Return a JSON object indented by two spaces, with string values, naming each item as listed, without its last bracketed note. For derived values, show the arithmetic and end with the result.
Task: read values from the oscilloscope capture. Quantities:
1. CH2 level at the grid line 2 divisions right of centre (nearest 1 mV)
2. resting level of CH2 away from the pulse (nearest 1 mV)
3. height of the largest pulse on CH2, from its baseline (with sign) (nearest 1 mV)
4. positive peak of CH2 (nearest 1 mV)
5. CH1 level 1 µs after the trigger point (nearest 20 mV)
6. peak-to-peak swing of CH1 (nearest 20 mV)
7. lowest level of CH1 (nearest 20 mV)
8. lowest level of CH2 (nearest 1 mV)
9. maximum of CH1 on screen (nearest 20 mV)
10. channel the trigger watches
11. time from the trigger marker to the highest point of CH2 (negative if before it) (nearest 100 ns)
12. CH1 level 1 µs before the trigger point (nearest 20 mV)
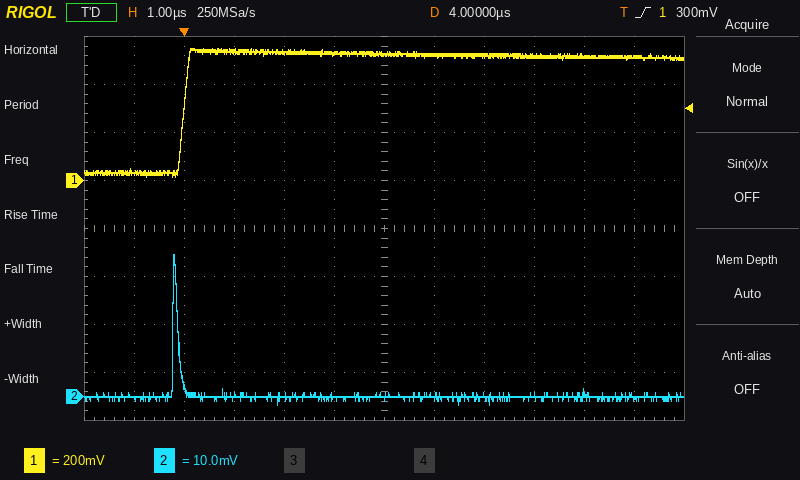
{
  "CH2 level at the grid line 2 divisions right of centre": "0 mV",
  "resting level of CH2 away from the pulse": "0 mV",
  "height of the largest pulse on CH2, from its baseline (with sign)": "30 mV − (0 mV) = +30 mV",
  "positive peak of CH2": "30 mV",
  "CH1 level 1 µs after the trigger point": "540 mV",
  "peak-to-peak swing of CH1": "560 mV − (20 mV) = 540 mV",
  "lowest level of CH1": "20 mV",
  "lowest level of CH2": "-2 mV",
  "maximum of CH1 on screen": "560 mV",
  "channel the trigger watches": "CH1",
  "time from the trigger marker to the highest point of CH2 (negative if before it)": "-200 ns",
  "CH1 level 1 µs before the trigger point": "40 mV"
}
